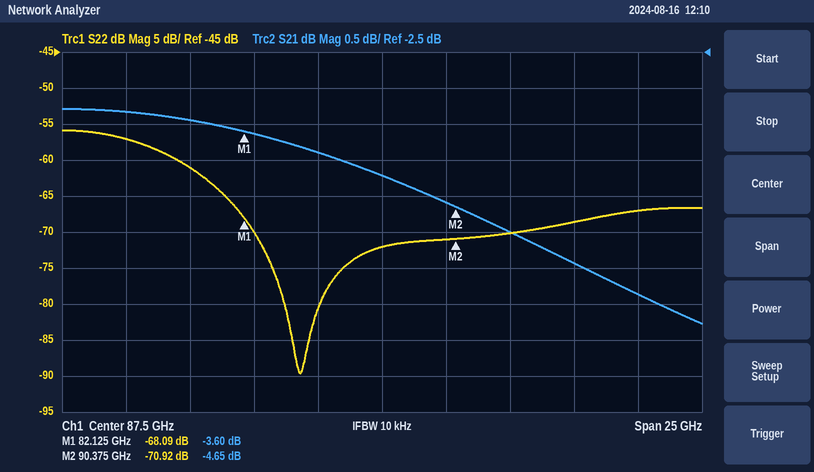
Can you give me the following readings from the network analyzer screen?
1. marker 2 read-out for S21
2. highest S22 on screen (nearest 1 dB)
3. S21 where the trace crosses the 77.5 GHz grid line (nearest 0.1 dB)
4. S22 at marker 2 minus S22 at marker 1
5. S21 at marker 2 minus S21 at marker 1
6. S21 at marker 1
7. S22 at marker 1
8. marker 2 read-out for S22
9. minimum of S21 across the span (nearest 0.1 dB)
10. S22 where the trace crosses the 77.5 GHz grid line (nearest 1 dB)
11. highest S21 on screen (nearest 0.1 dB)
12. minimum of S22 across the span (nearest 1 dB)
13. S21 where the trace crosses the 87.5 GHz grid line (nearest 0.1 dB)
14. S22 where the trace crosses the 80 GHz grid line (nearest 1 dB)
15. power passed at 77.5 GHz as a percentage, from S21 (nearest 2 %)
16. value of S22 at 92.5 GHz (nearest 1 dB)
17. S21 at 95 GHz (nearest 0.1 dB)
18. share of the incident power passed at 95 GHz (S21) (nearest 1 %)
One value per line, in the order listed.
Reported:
-4.65 dB
-56 dB
-3.3 dB
-2.83 dB
-1.05 dB
-3.60 dB
-68.09 dB
-70.92 dB
-6.3 dB
-57 dB
-3.3 dB
-90 dB
-4.2 dB
-61 dB
46 %
-70 dB
-5.4 dB
29 %
